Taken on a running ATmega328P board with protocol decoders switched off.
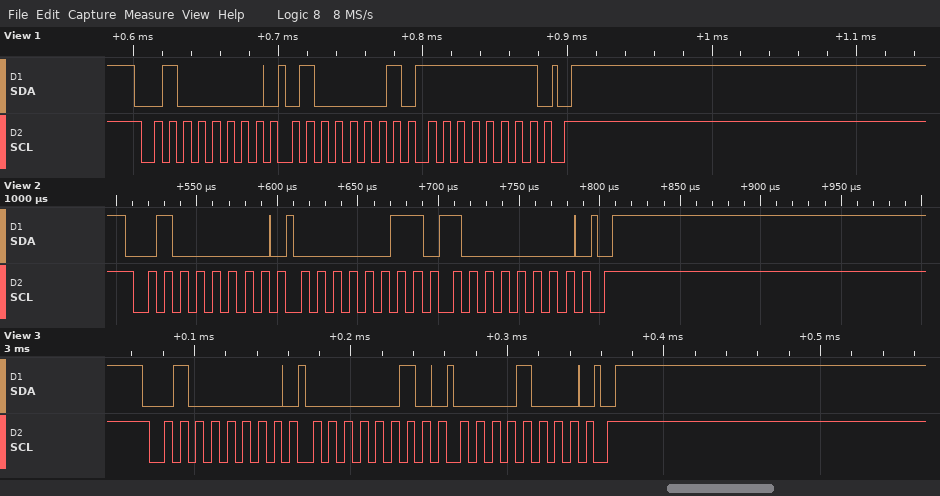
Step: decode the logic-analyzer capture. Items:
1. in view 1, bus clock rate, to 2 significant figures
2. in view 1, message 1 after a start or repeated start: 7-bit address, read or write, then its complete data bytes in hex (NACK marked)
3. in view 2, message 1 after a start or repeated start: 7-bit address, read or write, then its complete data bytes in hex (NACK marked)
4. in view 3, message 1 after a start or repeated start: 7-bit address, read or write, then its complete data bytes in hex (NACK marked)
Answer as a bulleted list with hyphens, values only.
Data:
- 100 kHz
- 0x20 write: 41 FF
- 0x20 write: 03 80
- 0x20 write: 02 08
